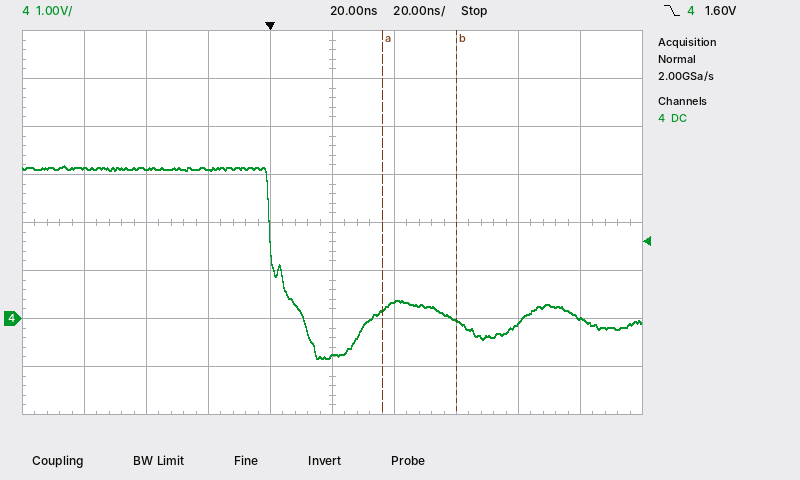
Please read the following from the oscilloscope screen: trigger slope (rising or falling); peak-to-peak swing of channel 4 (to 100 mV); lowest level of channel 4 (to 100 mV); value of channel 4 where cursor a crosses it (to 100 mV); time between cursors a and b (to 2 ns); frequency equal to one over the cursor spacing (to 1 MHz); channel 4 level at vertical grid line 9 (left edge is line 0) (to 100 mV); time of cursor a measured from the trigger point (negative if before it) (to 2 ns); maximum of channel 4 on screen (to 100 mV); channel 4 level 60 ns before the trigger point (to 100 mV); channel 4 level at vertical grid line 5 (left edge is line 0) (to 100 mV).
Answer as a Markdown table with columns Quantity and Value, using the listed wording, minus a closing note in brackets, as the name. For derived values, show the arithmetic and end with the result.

| Quantity | Value |
|---|---|
| trigger slope | falling |
| peak-to-peak swing of channel 4 | 3.2 V − (-800 mV) = 4.0 V |
| lowest level of channel 4 | -800 mV |
| value of channel 4 where cursor a crosses it | 200 mV |
| time between cursors a and b | 24 ns |
| frequency equal to one over the cursor spacing | 1 / 24 ns ≈ 42 MHz |
| channel 4 level at vertical grid line 9 (left edge is line 0) | 0.0 V |
| time of cursor a measured from the trigger point (negative if before it) | +36 ns |
| maximum of channel 4 on screen | 3.2 V |
| channel 4 level 60 ns before the trigger point | 3.1 V |
| channel 4 level at vertical grid line 5 (left edge is line 0) | -800 mV |
